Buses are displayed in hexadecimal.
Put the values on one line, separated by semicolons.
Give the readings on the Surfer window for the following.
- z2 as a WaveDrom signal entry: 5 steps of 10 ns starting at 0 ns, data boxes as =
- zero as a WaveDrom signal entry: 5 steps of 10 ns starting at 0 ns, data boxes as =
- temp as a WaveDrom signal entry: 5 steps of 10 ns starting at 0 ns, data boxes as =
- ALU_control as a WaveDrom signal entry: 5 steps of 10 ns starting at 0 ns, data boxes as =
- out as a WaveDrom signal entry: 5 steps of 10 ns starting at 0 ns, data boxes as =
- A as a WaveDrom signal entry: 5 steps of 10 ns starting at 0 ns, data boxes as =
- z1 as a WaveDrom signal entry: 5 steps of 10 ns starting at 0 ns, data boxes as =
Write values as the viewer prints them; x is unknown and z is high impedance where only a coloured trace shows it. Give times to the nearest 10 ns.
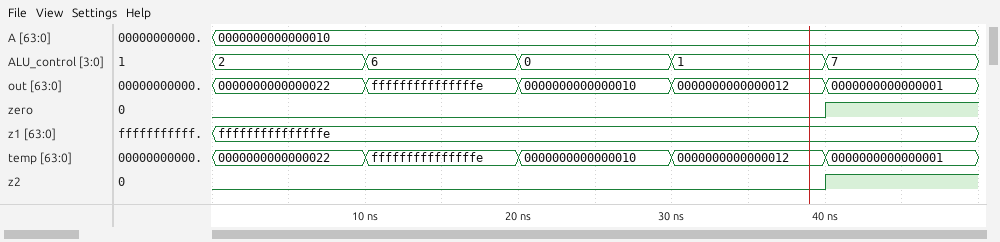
{name: 'z2', wave: '0...1'}; {name: 'zero', wave: '0...1'}; {name: 'temp', wave: '=====', data: '0000000000000022 fffffffffffffffe 0000000000000010 0000000000000012 0000000000000001'}; {name: 'ALU_control', wave: '=====', data: '2 6 0 1 7'}; {name: 'out', wave: '=====', data: '0000000000000022 fffffffffffffffe 0000000000000010 0000000000000012 0000000000000001'}; {name: 'A', wave: '=....', data: '0000000000000010'}; {name: 'z1', wave: '=....', data: 'fffffffffffffffe'}
